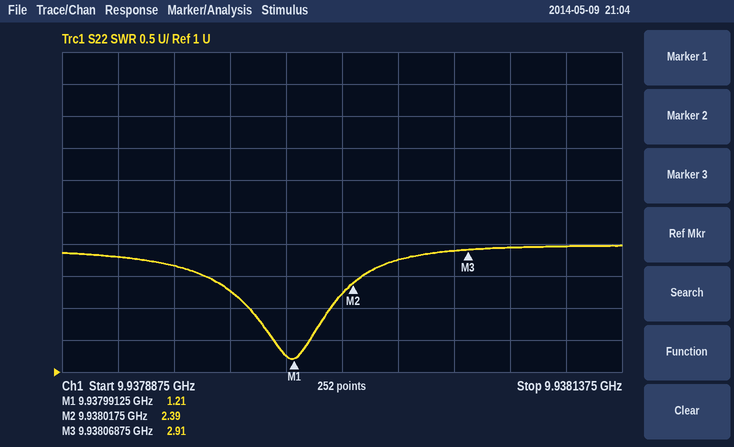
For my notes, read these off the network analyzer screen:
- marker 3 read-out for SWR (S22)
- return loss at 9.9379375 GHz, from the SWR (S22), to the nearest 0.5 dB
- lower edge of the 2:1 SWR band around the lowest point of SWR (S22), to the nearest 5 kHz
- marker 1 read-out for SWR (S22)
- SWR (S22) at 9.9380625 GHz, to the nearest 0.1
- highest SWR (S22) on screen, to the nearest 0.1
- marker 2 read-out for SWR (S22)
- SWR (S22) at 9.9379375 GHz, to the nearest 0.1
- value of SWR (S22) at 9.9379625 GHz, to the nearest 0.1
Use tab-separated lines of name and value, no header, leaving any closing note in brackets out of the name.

marker 3 read-out for SWR	2.91
return loss at 9.9379375 GHz, from the SWR (S22), to the nearest 0.5 dB	7.0 dB
lower edge of the 2:1 SWR band around the lowest point of SWR (S22), to the nearest 5 kHz	9.937970 GHz
marker 1 read-out for SWR	1.21
SWR (S22) at 9.9380625 GHz, to the nearest 0.1	2.9
highest SWR (S22) on screen, to the nearest 0.1	3.0
marker 2 read-out for SWR	2.39
SWR (S22) at 9.9379375 GHz, to the nearest 0.1	2.7
value of SWR (S22) at 9.9379625 GHz, to the nearest 0.1	2.3
